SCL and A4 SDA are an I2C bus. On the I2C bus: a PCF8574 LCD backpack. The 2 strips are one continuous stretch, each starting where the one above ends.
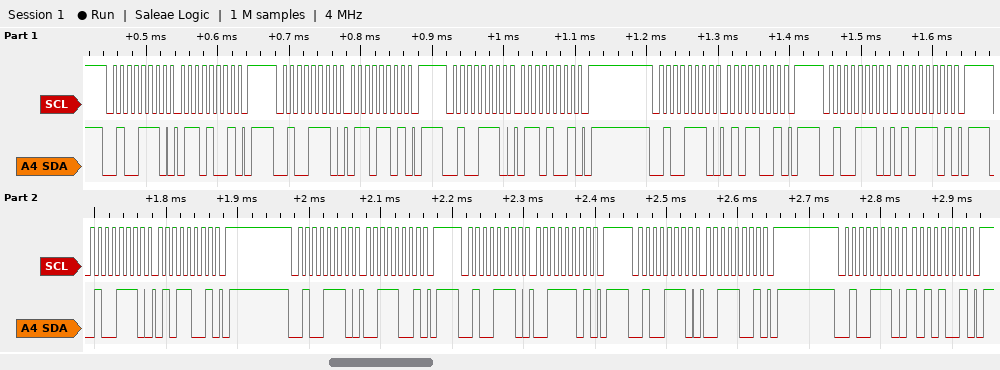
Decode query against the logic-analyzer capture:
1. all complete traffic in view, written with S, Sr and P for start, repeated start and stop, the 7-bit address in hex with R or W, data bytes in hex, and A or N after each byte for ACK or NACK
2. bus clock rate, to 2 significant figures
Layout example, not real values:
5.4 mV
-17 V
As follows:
S 27W A 69 A P S 27W A 6D A P S 27W A 69 A P S 27W A 59 A P S 27W A 5D A P S 27W A 59 A P S 27W A 39 A P S 27W A 3D A P S 27W A 39 A P S 27W A A9 A P
100 kHz
